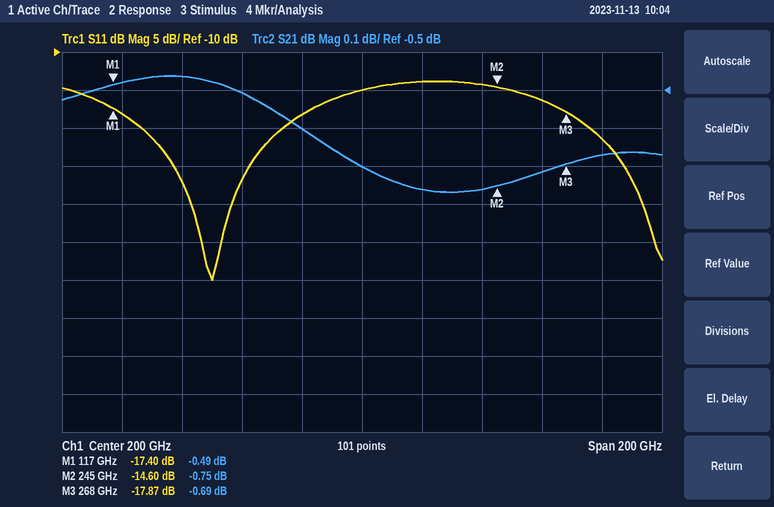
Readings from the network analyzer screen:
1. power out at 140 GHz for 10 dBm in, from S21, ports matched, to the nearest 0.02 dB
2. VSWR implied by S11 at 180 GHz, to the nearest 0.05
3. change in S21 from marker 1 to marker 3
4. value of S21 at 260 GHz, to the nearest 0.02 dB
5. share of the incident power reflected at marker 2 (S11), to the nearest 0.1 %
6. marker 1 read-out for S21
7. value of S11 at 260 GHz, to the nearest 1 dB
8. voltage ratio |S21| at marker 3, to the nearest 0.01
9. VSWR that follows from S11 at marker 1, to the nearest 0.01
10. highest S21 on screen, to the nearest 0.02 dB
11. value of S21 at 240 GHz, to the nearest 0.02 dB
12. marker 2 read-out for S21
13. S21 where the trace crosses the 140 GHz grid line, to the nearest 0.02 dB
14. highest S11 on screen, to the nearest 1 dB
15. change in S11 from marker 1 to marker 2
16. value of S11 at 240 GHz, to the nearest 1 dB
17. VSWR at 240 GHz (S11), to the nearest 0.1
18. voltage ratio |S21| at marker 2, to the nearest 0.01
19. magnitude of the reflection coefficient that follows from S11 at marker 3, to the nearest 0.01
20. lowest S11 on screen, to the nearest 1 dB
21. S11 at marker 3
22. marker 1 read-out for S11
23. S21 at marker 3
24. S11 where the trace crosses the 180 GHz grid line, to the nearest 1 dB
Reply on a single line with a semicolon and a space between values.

9.54 dBm; 1.30; -0.20 dB; -0.72 dB; 3.5 %; -0.49 dB; -16 dB; 0.92; 1.31; -0.46 dB; -0.76 dB; -0.75 dB; -0.46 dB; -14 dB; 2.80 dB; -14 dB; 1.5; 0.92; 0.13; -40 dB; -17.87 dB; -17.40 dB; -0.69 dB; -18 dB
